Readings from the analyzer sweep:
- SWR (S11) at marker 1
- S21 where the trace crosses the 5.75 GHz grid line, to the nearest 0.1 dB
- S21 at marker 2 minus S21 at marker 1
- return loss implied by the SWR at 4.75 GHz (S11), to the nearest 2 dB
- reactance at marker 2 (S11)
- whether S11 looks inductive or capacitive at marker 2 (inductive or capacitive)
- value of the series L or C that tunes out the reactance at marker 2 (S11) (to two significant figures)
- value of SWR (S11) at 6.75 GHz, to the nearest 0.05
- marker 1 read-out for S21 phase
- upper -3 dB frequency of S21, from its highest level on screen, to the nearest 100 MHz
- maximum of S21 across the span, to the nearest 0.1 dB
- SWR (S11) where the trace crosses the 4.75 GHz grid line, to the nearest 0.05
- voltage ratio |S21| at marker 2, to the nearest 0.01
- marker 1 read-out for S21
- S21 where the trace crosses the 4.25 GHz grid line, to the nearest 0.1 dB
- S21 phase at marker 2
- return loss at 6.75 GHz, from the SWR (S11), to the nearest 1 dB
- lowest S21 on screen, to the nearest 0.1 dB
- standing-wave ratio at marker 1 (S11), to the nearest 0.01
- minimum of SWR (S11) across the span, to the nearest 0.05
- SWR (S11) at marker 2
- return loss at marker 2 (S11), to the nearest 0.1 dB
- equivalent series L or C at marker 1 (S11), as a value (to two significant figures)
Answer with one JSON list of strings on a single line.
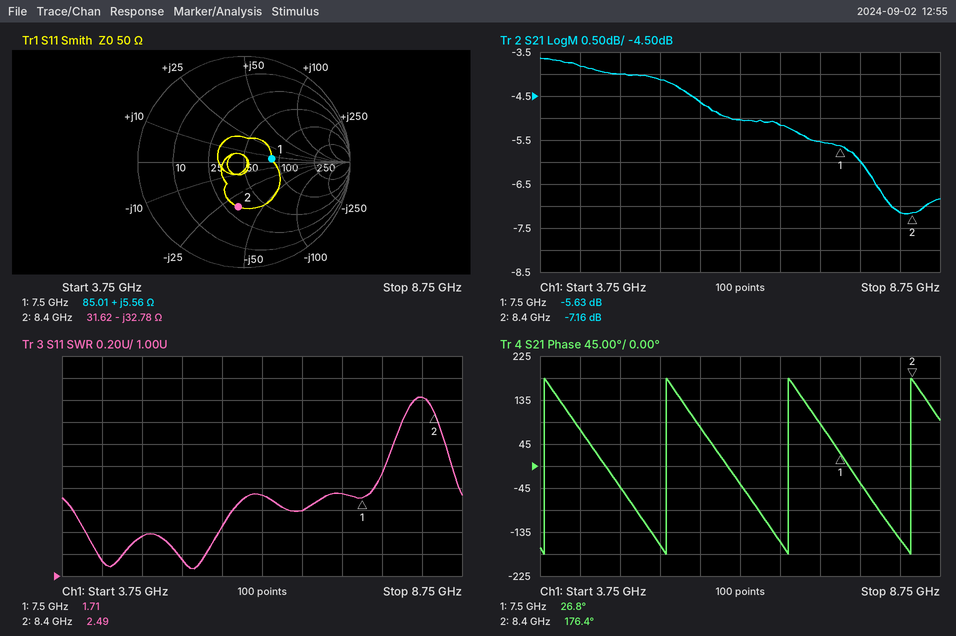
["1.71", "-4.6 dB", "-1.53 dB", "16 dB", "-32.78 Ω", "capacitive", "620 pH", "1.60", "26.8°", "8.0 GHz", "-3.6 dB", "1.35", "0.44", "-5.63 dB", "-3.8 dB", "176.4°", "13 dB", "-7.2 dB", "1.71", "1.05", "2.49", "7.4 dB", "120 pH"]
